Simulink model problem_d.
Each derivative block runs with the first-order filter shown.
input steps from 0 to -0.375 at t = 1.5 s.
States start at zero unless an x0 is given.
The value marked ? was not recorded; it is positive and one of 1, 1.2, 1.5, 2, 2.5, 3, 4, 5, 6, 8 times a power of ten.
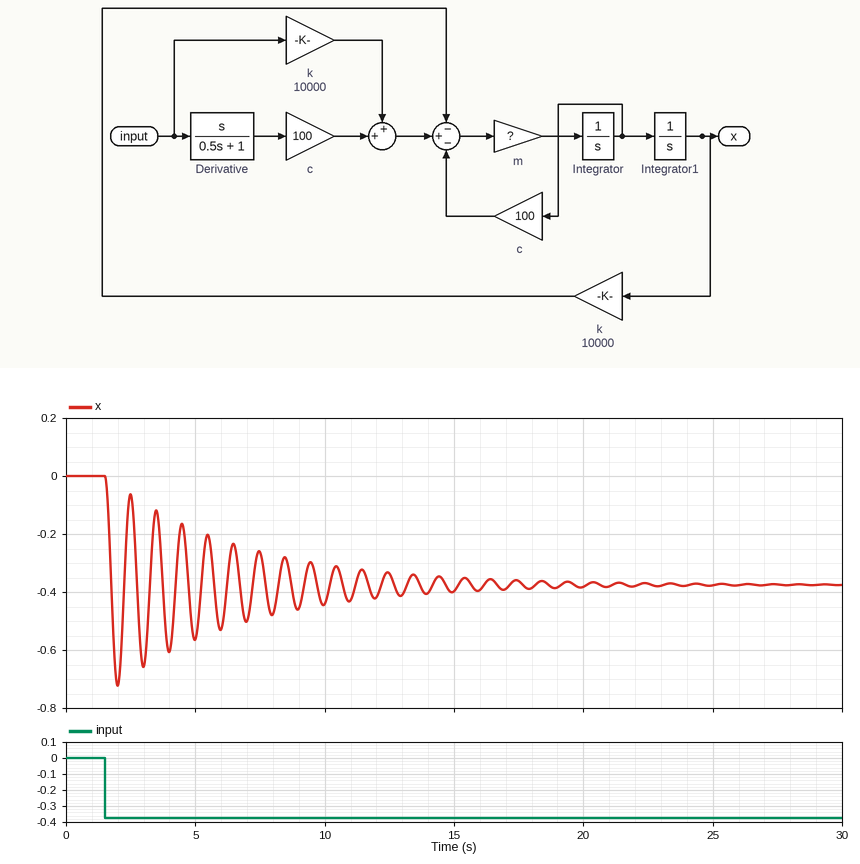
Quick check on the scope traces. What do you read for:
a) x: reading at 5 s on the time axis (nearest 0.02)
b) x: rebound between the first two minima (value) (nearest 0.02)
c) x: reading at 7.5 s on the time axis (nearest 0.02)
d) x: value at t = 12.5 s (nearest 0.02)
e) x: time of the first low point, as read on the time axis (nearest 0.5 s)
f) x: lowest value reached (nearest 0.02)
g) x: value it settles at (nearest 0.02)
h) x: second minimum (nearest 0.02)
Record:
-0.56
-0.06
-0.26
-0.34
2.0 s
-0.72
-0.38
-0.66
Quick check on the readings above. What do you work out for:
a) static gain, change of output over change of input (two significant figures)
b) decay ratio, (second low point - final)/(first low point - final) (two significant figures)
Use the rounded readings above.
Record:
1.0
0.82
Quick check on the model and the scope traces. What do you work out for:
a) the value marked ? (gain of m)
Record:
0.004
